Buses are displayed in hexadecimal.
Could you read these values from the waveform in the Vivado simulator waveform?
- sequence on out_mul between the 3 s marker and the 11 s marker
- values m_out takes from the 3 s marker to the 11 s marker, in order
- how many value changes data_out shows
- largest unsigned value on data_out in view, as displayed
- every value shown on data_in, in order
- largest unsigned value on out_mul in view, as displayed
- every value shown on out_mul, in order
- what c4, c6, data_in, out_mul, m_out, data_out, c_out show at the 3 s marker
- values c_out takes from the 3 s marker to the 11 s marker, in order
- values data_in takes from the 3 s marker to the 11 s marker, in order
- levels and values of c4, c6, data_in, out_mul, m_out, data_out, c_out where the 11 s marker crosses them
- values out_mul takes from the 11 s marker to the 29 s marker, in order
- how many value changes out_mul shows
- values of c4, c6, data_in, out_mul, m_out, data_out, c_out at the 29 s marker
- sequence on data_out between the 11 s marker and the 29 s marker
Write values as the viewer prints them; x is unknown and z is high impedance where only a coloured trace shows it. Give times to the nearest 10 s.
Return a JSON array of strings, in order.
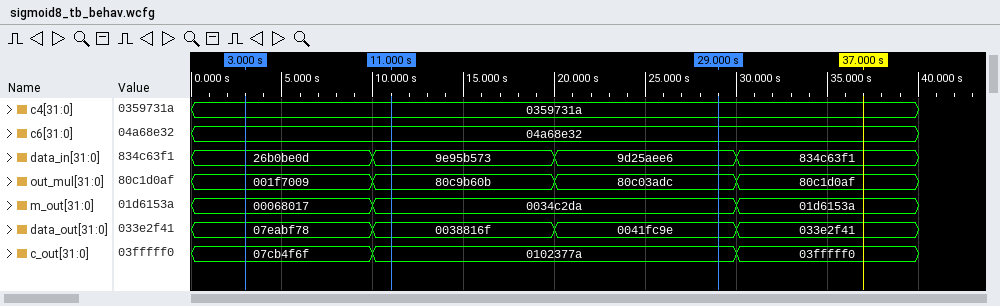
["001f7009, 80c9b60b", "00068017, 0034c2da", "3", "07eabf78", "26b0be0d, 9e95b573, 9d25aee6, 834c63f1", "80c9b60b", "001f7009, 80c9b60b, 80c03adc, 80c1d0af", "c4=0359731a, c6=04a68e32, data_in=26b0be0d, out_mul=001f7009, m_out=00068017, data_out=07eabf78, c_out=07cb4f6f", "07cb4f6f, 0102377a", "26b0be0d, 9e95b573", "c4=0359731a, c6=04a68e32, data_in=9e95b573, out_mul=80c9b60b, m_out=0034c2da, data_out=0038816f, c_out=0102377a", "80c9b60b, 80c03adc", "3", "c4=0359731a, c6=04a68e32, data_in=9d25aee6, out_mul=80c03adc, m_out=0034c2da, data_out=0041fc9e, c_out=0102377a", "0038816f, 0041fc9e"]
